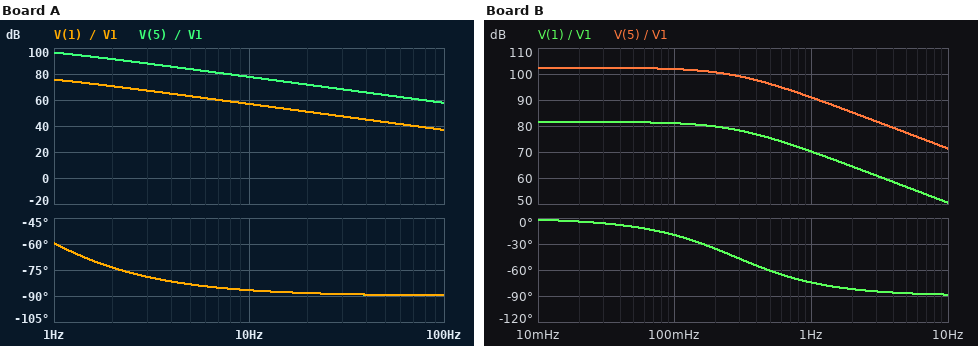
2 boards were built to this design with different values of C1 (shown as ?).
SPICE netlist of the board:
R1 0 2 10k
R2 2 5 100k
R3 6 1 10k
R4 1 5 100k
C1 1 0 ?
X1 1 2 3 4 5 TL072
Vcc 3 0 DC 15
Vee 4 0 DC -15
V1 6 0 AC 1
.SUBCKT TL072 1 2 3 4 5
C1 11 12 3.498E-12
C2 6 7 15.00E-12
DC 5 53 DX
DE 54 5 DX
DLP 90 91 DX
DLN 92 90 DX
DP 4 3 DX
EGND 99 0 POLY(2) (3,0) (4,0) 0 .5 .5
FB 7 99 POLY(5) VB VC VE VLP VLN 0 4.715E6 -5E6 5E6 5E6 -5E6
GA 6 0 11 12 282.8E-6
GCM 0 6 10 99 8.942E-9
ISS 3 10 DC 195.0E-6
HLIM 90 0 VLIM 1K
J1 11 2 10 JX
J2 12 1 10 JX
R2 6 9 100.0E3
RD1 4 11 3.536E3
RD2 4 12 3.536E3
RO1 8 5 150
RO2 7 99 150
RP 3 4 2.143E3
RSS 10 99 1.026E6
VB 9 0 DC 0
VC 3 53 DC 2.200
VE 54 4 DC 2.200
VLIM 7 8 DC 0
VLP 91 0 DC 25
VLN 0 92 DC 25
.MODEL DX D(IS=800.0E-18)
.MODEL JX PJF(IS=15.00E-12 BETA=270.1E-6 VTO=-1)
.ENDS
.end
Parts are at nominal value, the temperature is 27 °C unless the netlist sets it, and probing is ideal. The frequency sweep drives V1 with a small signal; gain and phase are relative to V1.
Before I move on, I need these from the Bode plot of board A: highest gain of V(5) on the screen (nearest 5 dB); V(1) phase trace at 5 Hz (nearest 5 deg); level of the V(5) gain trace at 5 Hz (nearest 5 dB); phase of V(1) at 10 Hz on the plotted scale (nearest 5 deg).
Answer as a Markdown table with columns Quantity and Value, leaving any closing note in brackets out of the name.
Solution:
| Quantity | Value |
|---|---|
| highest gain of V(5) on the screen | 95 dB |
| V(1) phase trace at 5 Hz | -85 deg |
| level of the V(5) gain trace at 5 Hz | 85 dB |
| phase of V(1) at 10 Hz on the plotted scale | -85 deg |
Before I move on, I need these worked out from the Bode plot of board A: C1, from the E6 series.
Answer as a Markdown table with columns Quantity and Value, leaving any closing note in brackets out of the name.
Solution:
| Quantity | Value |
|---|---|
| C1, from the E6 series | 2.2 nF |
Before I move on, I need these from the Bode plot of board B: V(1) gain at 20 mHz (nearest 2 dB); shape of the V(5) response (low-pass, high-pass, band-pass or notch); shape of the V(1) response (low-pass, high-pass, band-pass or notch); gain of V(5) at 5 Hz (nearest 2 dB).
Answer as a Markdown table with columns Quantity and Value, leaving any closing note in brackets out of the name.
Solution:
| Quantity | Value |
|---|---|
| V(1) gain at 20 mHz | 82 dB |
| shape of the V(5) response | low-pass |
| shape of the V(1) response | low-pass |
| gain of V(5) at 5 Hz | 78 dB |
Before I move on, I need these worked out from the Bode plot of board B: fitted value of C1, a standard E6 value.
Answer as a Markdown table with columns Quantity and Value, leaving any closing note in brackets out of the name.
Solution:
| Quantity | Value |
|---|---|
| fitted value of C1, a standard E6 value | 4.7 nF |
